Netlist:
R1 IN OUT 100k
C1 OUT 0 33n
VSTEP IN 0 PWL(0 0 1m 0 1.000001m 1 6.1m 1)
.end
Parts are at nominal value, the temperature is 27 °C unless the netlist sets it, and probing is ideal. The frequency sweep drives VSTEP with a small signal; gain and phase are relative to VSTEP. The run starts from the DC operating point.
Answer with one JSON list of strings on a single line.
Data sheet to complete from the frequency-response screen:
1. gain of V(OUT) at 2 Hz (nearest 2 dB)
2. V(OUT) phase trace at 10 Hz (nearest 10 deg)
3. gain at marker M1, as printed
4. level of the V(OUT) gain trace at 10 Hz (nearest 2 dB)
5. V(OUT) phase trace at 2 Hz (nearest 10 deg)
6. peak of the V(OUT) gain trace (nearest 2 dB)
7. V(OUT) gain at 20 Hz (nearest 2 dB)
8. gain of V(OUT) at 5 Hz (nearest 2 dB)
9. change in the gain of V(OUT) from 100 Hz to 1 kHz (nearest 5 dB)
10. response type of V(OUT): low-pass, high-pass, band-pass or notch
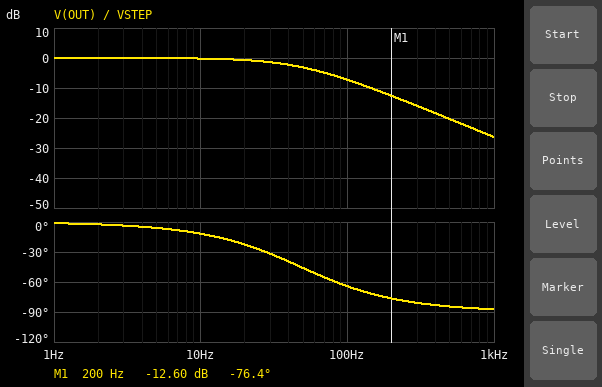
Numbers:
["0 dB", "-10 deg", "-12.60 dB", "0 dB", "0 deg", "0 dB", "0 dB", "0 dB", "-20 dB", "low-pass"]
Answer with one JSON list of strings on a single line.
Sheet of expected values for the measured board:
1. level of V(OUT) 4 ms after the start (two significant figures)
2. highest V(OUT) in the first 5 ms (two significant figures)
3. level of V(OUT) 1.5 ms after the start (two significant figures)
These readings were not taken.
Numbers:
["600 mV", "700 mV", "140 mV"]
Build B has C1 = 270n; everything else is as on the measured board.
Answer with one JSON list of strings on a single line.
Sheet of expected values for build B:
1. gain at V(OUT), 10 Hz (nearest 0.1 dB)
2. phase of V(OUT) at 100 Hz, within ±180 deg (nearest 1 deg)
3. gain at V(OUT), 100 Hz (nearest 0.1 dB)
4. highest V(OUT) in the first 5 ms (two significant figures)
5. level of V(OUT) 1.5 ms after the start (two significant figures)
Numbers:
["-5.9 dB", "-87 deg", "-24.6 dB", "140 mV", "18 mV"]
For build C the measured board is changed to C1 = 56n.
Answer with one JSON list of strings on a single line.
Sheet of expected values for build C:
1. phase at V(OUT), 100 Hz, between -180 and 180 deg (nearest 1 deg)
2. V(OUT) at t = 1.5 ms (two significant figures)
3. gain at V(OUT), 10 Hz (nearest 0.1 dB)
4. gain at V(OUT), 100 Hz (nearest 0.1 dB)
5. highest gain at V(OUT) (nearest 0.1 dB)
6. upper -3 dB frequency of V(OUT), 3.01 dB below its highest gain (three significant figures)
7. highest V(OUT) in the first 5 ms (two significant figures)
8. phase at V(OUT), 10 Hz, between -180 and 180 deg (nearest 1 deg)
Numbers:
["-74 deg", "85 mV", "-0.5 dB", "-11.3 dB", "0 dB", "28.4 Hz", "510 mV", "-19 deg"]
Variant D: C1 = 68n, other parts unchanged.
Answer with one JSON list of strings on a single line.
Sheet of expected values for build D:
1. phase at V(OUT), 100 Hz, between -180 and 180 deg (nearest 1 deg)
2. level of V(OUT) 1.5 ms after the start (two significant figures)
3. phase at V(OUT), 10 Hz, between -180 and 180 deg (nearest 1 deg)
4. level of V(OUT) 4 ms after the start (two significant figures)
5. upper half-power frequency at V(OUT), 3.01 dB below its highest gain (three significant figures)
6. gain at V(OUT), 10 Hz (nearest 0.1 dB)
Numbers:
["-77 deg", "71 mV", "-23 deg", "360 mV", "23.4 Hz", "-0.7 dB"]
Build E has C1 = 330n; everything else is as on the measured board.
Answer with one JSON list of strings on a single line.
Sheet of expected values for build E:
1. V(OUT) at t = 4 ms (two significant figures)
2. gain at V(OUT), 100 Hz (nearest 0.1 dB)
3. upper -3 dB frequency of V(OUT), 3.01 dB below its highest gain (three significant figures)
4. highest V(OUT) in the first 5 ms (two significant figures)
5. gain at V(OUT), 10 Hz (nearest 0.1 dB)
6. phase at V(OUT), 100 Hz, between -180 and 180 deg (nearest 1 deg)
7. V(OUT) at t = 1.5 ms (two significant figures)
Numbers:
["87 mV", "-26.3 dB", "4.82 Hz", "110 mV", "-7.2 dB", "-87 deg", "15 mV"]
